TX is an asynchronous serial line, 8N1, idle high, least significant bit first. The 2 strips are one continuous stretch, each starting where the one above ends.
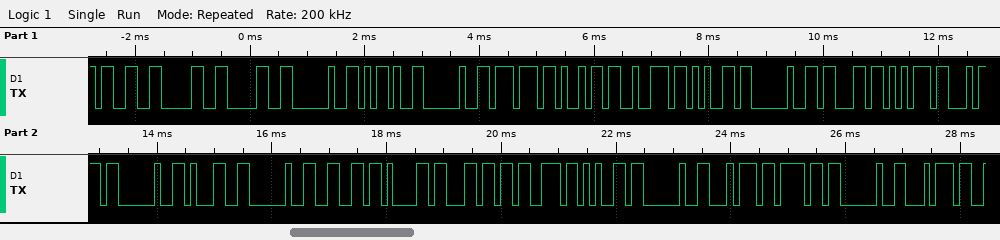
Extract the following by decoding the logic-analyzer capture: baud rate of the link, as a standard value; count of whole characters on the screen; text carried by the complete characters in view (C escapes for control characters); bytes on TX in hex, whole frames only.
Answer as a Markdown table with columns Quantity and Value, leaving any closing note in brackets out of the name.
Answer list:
| Quantity | Value |
|---|---|
| baud rate of the link, as a standard value | 9600 baud |
| count of whole characters on the screen | 27 |
| text carried by the complete characters in view | "300 - wire cut 1 false to t" |
| bytes on TX in hex, whole frames only | 33 30 30 20 2D 20 77 69 72 65 20 63 75 74 20 31 20 66 61 6C 73 65 20 74 6F 20 74 |
